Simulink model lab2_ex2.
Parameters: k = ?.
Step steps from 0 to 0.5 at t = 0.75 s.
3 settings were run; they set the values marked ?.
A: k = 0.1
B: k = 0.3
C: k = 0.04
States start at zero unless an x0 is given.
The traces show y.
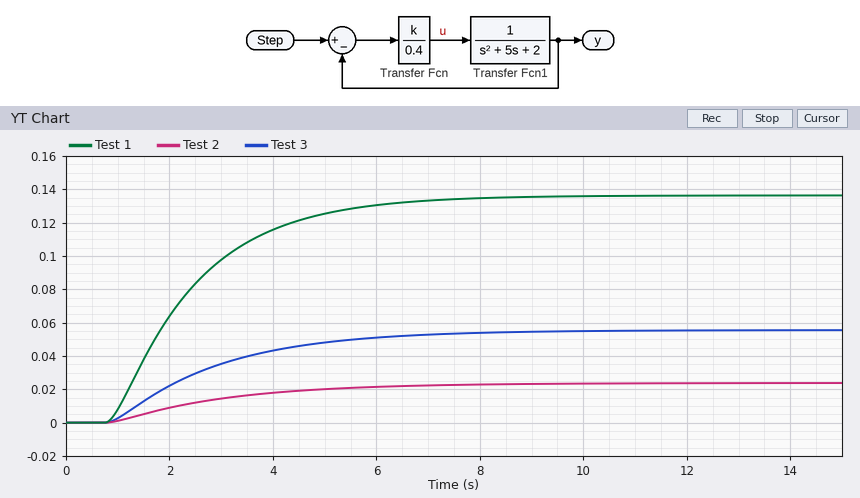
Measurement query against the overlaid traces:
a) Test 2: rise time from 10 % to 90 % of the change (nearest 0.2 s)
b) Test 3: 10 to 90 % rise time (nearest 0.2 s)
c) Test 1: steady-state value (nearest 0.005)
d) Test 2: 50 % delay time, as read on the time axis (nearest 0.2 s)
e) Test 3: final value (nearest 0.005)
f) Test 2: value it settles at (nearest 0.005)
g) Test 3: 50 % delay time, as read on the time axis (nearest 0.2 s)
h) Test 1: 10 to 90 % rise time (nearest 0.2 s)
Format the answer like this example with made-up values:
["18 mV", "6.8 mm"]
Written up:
["4.8 s", "4.4 s", "0.135", "2.4 s", "0.055", "0.025", "2.4 s", "3.6 s"]
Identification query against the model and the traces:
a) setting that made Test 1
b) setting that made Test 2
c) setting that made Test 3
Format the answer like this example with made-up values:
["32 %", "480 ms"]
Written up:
["B", "C", "A"]
